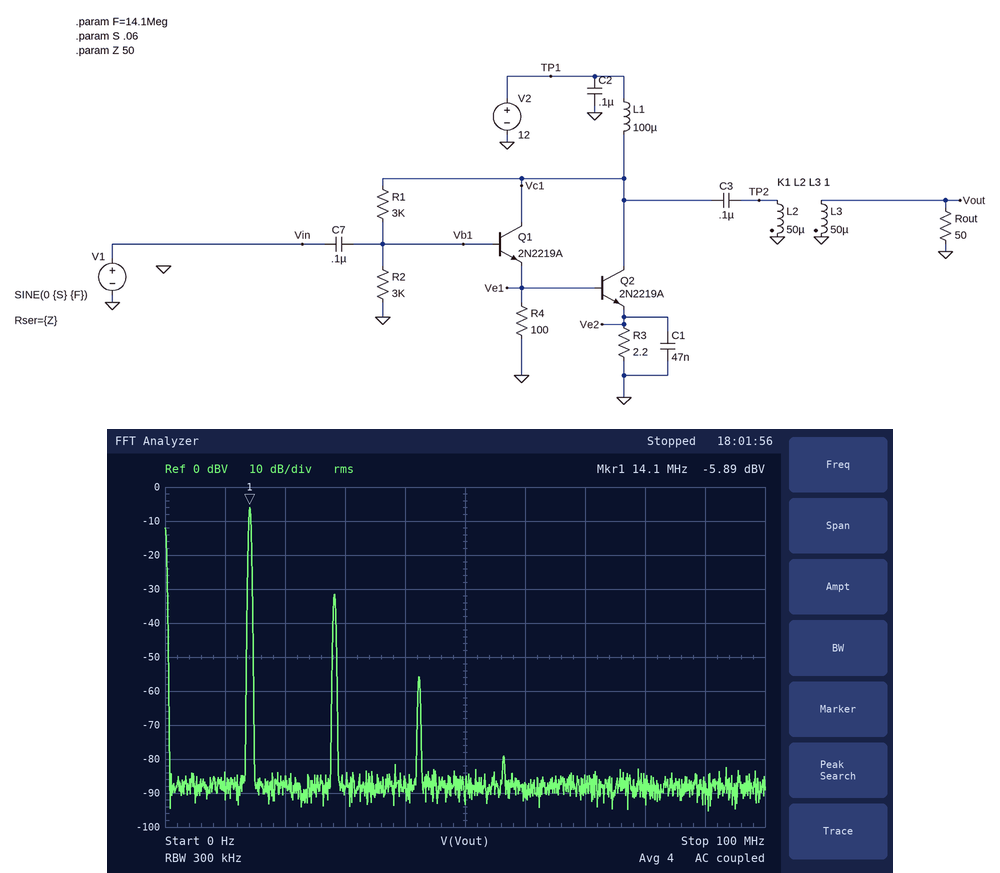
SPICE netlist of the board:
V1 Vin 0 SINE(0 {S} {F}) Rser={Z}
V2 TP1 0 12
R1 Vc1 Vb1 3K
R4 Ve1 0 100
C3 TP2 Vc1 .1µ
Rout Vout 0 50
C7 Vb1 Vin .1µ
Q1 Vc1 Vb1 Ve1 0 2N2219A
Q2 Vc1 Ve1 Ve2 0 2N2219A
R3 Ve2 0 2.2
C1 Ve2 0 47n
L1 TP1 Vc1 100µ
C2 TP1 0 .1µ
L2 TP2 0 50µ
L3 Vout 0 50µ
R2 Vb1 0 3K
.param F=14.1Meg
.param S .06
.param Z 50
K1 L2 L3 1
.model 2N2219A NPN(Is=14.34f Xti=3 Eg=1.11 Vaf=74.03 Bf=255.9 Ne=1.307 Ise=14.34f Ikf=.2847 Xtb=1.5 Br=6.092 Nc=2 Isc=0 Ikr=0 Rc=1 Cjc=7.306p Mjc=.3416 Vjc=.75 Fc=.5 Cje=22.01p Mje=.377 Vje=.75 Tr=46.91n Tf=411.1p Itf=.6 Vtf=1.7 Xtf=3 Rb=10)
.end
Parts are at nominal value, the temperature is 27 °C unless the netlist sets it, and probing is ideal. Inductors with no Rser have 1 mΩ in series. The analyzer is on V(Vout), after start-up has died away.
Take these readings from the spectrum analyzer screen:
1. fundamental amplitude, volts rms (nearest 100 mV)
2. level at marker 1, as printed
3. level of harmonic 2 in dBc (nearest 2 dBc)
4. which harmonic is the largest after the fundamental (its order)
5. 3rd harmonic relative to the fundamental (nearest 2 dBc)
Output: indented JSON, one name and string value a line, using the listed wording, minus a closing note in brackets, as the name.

{
  "fundamental amplitude, volts rms": "500 mV",
  "level at marker 1, as printed": "-5.89 dBV",
  "level of harmonic 2 in dBc": "-26 dBc",
  "which harmonic is the largest after the fundamental": "2",
  "3rd harmonic relative to the fundamental": "-50 dBc"
}
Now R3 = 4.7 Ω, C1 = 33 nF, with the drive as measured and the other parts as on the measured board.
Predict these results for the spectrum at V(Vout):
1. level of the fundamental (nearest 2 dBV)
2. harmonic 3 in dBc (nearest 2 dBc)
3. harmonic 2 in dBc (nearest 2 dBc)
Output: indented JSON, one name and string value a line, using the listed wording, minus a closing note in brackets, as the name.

{
  "level of the fundamental": "-2 dBV",
  "harmonic 3 in dBc": "-48 dBc",
  "harmonic 2 in dBc": "-24 dBc"
}
